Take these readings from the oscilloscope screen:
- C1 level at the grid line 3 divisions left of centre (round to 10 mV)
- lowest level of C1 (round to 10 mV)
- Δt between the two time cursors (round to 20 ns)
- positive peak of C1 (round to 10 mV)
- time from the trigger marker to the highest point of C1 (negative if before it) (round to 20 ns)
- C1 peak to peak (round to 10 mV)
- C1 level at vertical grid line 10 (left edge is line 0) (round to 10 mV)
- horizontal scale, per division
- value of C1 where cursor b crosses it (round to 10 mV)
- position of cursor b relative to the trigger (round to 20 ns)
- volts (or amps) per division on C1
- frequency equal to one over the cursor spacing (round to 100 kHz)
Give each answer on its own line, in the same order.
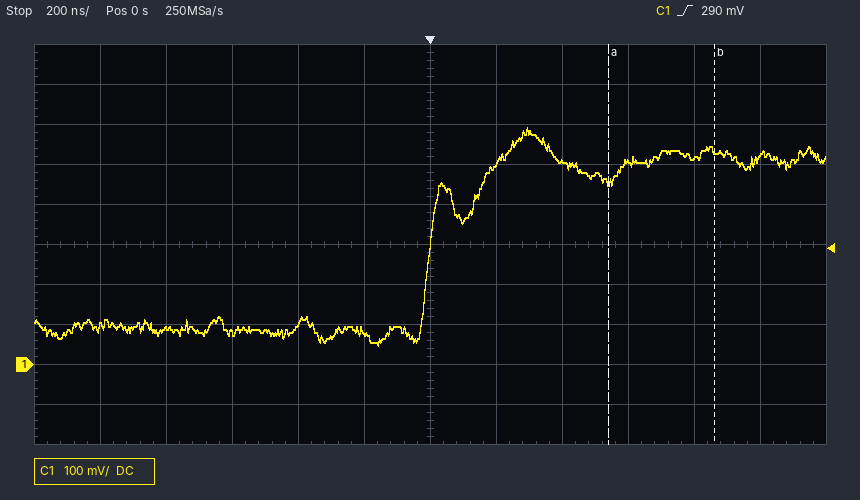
80 mV
50 mV
320 ns
590 mV
+300 ns
540 mV
520 mV
200 ns
540 mV
+860 ns
100 mV
3.1 MHz
